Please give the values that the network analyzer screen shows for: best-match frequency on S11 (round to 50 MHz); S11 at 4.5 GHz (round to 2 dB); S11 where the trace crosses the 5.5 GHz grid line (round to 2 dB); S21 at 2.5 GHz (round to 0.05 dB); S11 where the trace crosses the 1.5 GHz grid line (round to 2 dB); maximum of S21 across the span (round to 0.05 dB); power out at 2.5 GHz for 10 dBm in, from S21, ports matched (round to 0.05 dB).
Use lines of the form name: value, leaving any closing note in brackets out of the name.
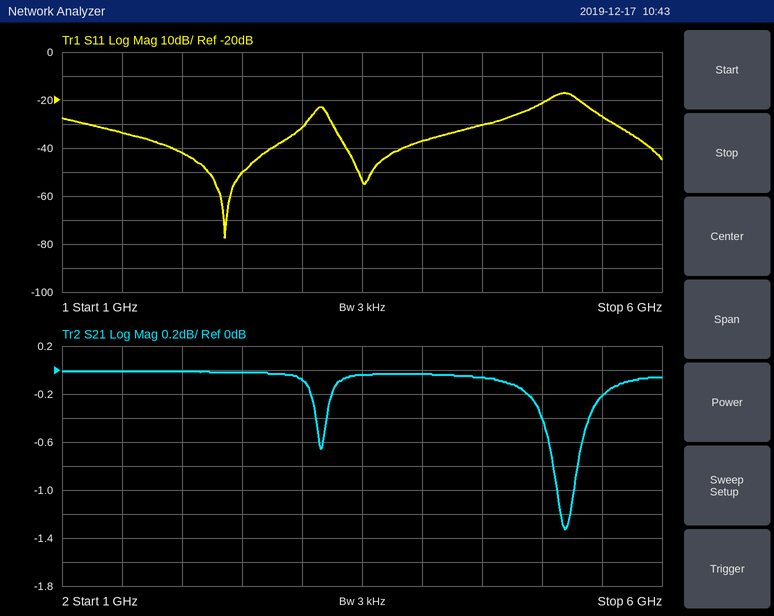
best-match frequency on S11: 2.35 GHz
S11 at 4.5 GHz: -30 dB
S11 where the trace crosses the 5.5 GHz grid line: -26 dB
S21 at 2.5 GHz: 0.00 dB
S11 where the trace crosses the 1.5 GHz grid line: -34 dB
maximum of S21 across the span: 0.00 dB
power out at 2.5 GHz for 10 dBm in, from S21, ports matched: 10.00 dBm
